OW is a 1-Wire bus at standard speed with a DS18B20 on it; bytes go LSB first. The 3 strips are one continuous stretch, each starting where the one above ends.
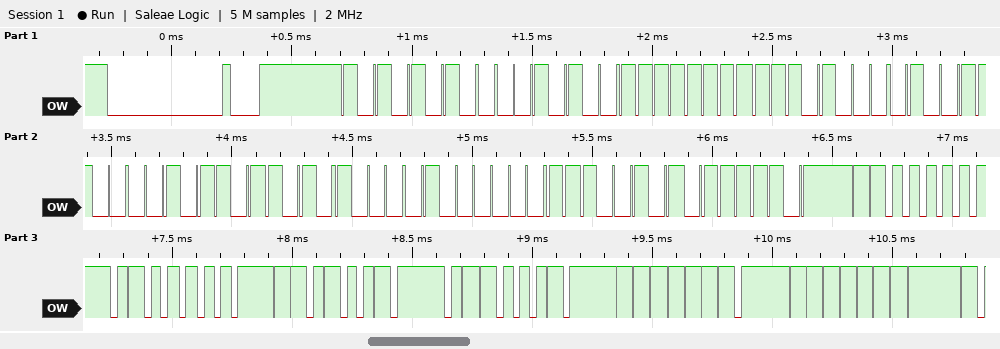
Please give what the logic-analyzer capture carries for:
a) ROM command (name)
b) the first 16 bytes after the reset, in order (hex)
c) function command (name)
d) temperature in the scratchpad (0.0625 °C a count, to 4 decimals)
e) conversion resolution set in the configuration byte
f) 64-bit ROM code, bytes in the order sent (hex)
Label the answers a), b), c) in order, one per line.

a) Match ROM
b) 55 28 FF 17 32 B4 15 02 A7 BE 03 02 4B 46 7F FF
c) Read Scratchpad
d) 32.1875 °C
e) 12 bits
f) 28 FF 17 32 B4 15 02 A7
